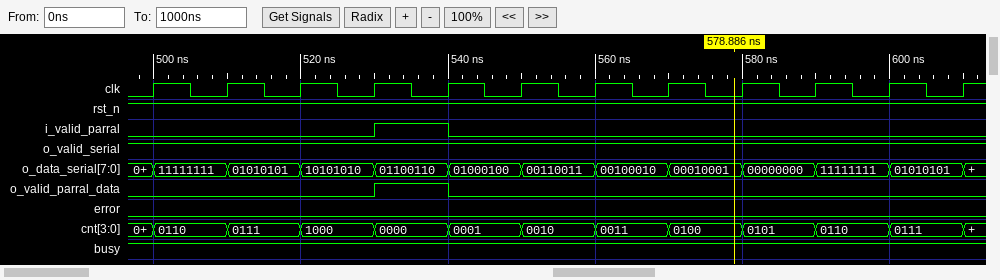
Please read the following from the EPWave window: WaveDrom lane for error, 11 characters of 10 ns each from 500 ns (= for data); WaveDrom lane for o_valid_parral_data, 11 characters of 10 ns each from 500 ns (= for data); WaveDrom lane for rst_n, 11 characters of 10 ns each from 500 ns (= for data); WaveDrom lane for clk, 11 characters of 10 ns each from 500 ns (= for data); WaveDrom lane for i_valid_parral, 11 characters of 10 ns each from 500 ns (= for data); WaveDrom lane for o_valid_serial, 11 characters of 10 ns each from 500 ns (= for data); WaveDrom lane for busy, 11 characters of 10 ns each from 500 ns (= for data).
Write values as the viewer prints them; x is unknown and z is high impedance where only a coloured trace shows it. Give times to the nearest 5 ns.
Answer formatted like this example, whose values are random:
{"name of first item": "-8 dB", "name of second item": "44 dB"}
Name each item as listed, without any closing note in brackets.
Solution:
{"WaveDrom lane for error, 11 characters of 10 ns each from 500 ns": "{name: 'error', wave: '0..........'}", "WaveDrom lane for o_valid_parral_data, 11 characters of 10 ns each from 500 ns": "{name: 'o_valid_parral_data', wave: '0..10......'}", "WaveDrom lane for rst_n, 11 characters of 10 ns each from 500 ns": "{name: 'rst_n', wave: '1..........'}", "WaveDrom lane for clk, 11 characters of 10 ns each from 500 ns": "{name: 'clk', wave: 'p..........'}", "WaveDrom lane for i_valid_parral, 11 characters of 10 ns each from 500 ns": "{name: 'i_valid_parral', wave: '0..10......'}", "WaveDrom lane for o_valid_serial, 11 characters of 10 ns each from 500 ns": "{name: 'o_valid_serial', wave: '1..........'}", "WaveDrom lane for busy, 11 characters of 10 ns each from 500 ns": "{name: 'busy', wave: '1..........'}"}
